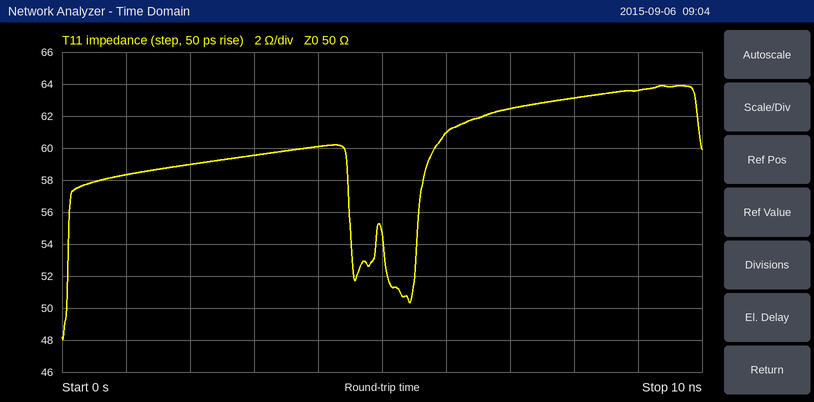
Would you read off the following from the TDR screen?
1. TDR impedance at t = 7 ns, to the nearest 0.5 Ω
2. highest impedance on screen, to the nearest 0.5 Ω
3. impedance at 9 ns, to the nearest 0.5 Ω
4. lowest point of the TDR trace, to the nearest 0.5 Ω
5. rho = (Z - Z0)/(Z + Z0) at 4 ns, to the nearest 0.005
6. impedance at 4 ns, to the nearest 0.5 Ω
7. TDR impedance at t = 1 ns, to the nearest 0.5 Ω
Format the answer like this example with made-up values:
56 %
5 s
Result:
62.5 Ω
64.0 Ω
63.5 Ω
48.0 Ω
+0.090
60.0 Ω
58.5 Ω
